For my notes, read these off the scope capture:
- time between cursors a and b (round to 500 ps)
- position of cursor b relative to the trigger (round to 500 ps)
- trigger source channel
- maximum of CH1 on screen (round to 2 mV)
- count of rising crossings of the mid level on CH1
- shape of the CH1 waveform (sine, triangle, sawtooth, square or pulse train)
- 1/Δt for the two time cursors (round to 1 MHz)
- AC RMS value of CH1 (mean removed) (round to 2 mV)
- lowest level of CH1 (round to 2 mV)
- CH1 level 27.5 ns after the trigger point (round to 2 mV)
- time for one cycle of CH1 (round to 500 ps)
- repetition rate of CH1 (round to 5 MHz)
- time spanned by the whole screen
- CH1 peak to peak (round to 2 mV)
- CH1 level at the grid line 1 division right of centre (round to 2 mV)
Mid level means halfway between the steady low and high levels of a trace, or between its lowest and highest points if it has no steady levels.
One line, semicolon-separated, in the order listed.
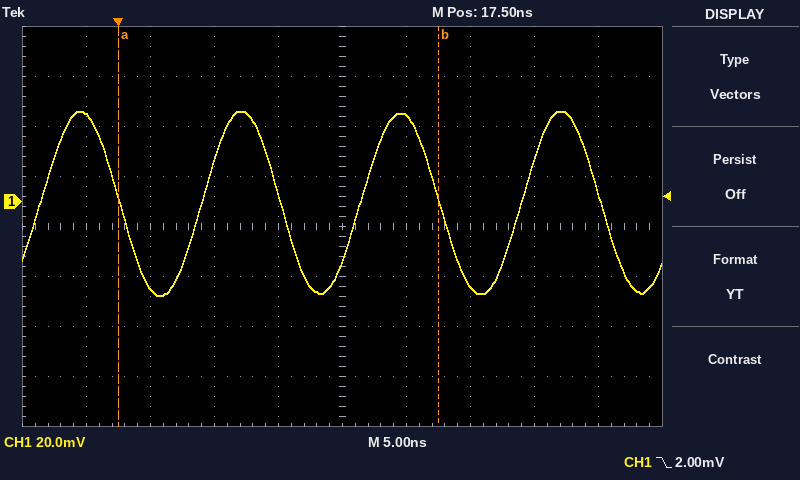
25.0 ns; +25.0 ns; CH1; 36 mV; 4; sine; 40 MHz; 26 mV; -38 mV; -34 mV; 12.5 ns; 80 MHz; 50 ns; 74 mV; 34 mV
